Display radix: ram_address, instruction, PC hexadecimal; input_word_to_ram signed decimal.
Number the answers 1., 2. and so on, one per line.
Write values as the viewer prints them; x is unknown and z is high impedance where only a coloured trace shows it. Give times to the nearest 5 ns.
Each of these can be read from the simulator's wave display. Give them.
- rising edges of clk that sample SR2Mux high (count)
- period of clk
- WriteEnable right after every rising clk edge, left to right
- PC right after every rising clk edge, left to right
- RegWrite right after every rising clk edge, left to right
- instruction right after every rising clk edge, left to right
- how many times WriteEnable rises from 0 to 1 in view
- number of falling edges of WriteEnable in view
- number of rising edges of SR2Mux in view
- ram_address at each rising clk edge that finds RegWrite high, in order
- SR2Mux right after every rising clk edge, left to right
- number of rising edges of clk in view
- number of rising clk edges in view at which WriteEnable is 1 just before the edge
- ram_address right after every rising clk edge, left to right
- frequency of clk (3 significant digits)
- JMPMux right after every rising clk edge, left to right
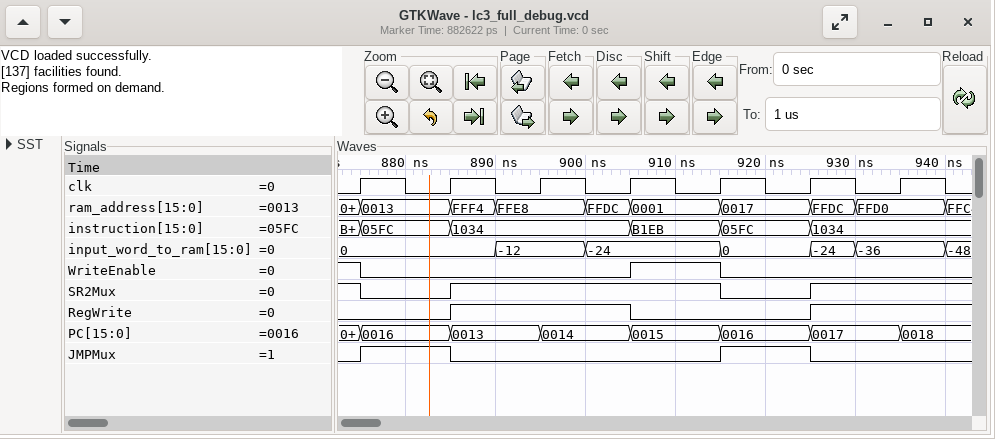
1. 5
2. 10 ns
3. 0 0 0 1 0 0 0
4. 0016, 0013, 0014, 0015, 0016, 0017, 0018
5. 0 1 1 0 0 1 1
6. 05FC, 1034, 1034, B1EB, 05FC, 1034, 1034
7. 1
8. 2
9. 2
10. FFE8, FFDC, FFD0
11. 0 1 1 1 0 1 1
12. 7
13. 2
14. 0013, FFF4, FFE8, 0001, 0017, FFDC, FFD0
15. 100 MHz
16. 1 0 0 0 1 0 0
